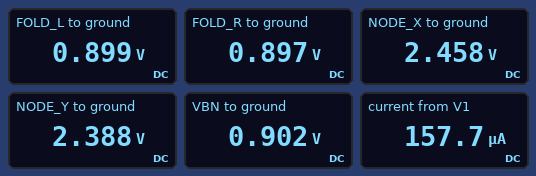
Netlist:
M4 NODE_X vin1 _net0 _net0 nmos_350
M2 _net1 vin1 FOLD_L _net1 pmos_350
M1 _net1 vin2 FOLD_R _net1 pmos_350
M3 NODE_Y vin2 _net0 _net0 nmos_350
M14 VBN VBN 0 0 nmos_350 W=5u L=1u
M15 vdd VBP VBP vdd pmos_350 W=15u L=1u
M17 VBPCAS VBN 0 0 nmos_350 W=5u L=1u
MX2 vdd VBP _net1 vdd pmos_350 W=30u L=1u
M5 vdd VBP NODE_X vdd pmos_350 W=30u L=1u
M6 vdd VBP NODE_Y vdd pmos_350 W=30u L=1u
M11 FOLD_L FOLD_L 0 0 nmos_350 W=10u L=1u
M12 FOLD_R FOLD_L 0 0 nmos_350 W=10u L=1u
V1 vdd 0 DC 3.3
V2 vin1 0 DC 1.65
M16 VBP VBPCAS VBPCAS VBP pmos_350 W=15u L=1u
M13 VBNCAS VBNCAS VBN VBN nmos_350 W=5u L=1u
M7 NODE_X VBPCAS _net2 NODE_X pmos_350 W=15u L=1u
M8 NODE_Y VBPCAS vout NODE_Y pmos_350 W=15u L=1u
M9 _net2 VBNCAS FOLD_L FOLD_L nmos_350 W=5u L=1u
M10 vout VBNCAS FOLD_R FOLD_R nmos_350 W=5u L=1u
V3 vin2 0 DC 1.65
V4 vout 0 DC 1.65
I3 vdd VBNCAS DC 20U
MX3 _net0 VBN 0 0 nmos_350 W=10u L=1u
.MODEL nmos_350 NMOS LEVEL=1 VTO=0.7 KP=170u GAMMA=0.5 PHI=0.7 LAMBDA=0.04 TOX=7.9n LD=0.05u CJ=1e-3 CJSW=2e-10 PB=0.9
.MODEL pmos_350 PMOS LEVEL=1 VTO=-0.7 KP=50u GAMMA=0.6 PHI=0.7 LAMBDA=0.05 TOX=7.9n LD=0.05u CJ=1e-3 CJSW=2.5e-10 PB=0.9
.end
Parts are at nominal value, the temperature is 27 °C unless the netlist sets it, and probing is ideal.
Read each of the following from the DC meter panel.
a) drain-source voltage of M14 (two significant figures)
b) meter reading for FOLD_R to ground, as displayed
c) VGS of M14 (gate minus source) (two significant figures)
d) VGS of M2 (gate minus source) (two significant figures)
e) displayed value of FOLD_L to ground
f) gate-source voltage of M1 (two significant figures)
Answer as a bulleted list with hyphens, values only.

- 900 mV
- 0.897 V
- 900 mV
- 750 mV
- 0.899 V
- 750 mV
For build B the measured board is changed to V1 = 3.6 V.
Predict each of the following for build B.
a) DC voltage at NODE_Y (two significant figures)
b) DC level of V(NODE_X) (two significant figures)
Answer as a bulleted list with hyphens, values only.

- 2.7 V
- 3.1 V
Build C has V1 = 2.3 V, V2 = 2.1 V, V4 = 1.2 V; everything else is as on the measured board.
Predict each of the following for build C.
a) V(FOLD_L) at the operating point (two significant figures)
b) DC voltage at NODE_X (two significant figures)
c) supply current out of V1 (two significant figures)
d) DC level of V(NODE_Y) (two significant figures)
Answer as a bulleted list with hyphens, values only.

- 760 mV
- 1.3 V
- 120 µA
- 1.5 V
